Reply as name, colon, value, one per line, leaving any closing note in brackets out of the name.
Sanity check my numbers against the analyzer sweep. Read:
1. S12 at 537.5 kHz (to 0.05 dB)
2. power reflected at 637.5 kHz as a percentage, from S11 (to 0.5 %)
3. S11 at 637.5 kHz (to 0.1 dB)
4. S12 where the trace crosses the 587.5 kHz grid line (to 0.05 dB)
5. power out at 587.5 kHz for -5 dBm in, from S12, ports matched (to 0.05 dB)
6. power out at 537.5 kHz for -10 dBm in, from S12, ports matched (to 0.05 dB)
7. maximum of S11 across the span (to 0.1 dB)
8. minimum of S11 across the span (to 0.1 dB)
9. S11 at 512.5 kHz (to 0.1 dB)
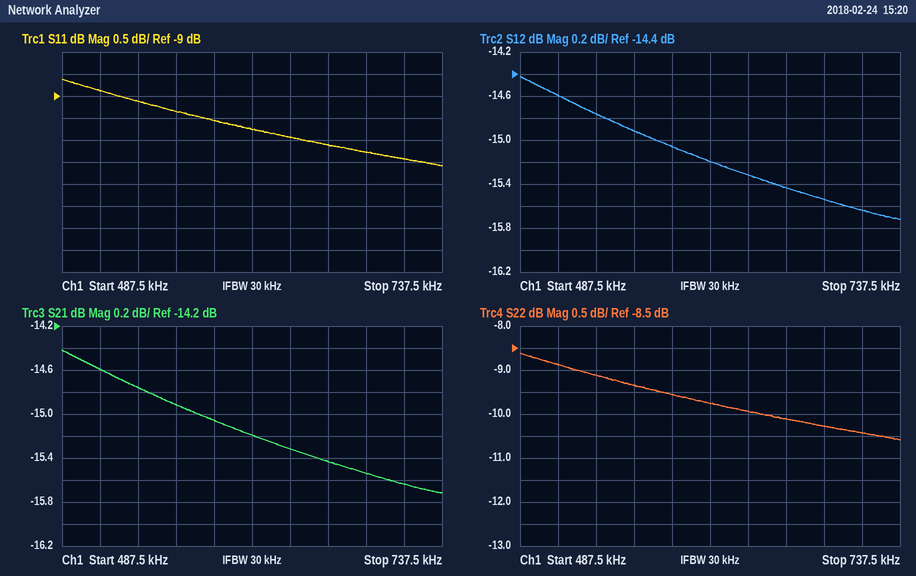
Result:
S12 at 537.5 kHz: -14.75 dB
power reflected at 637.5 kHz as a percentage, from S11: 10.0 %
S11 at 637.5 kHz: -9.9 dB
S12 where the trace crosses the 587.5 kHz grid line: -15.05 dB
power out at 587.5 kHz for -5 dBm in, from S12, ports matched: -20.05 dBm
power out at 537.5 kHz for -10 dBm in, from S12, ports matched: -24.75 dBm
maximum of S11 across the span: -8.6 dB
minimum of S11 across the span: -10.6 dB
S11 at 512.5 kHz: -8.9 dB
